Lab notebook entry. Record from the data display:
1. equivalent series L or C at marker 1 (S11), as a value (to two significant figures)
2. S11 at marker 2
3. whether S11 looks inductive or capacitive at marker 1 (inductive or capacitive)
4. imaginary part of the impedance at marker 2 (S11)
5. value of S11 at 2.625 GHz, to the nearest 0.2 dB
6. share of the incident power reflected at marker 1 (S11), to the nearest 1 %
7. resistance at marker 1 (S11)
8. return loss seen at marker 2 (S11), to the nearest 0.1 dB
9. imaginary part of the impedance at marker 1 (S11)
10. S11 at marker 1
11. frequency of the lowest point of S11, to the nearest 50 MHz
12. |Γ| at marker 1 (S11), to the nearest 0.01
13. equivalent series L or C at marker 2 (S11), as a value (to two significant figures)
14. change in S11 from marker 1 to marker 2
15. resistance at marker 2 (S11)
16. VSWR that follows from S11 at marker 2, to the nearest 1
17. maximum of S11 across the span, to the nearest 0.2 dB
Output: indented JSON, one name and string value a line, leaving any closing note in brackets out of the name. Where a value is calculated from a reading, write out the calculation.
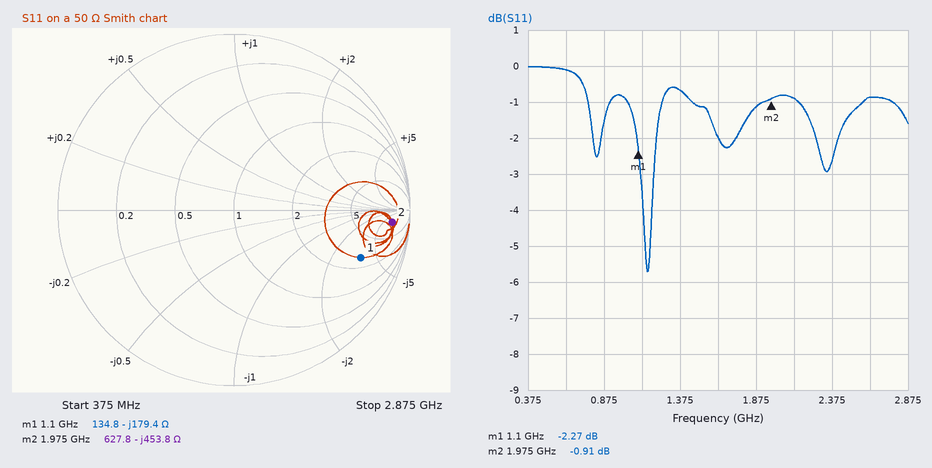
{
  "equivalent series L or C at marker 1 (S11), as a value": "C = 1/(2π × 1.1 GHz × 179.4 Ω) ≈ 807 fF, so 810 fF to two significant figures",
  "S11 at marker 2": "-0.91 dB",
  "whether S11 looks inductive or capacitive at marker 1": "capacitive",
  "imaginary part of the impedance at marker 2": "-453.8 Ω",
  "value of S11 at 2.625 GHz, to the nearest 0.2 dB": "-0.8 dB",
  "share of the incident power reflected at marker 1 (S11), to the nearest 1 %": "10^(-2.27/10) ≈ 59 %",
  "resistance at marker 1": "134.8 Ω",
  "return loss seen at marker 2 (S11), to the nearest 0.1 dB": "0.9 dB",
  "imaginary part of the impedance at marker 1": "-179.4 Ω",
  "S11 at marker 1": "-2.27 dB",
  "frequency of the lowest point of S11, to the nearest 50 MHz": "1.15 GHz",
  "|Γ| at marker 1 (S11), to the nearest 0.01": "0.77",
  "equivalent series L or C at marker 2 (S11), as a value": "C = 1/(2π × 1.975 GHz × 453.8 Ω) ≈ 178 fF, so 180 fF to two significant figures",
  "change in S11 from marker 1 to marker 2": "-0.91 − (-2.27) = 1.36 dB",
  "resistance at marker 2": "627.8 Ω",
  "VSWR that follows from S11 at marker 2, to the nearest 1": "(1 + 0.9005)/(1 − 0.9005) ≈ 19",
  "maximum of S11 across the span, to the nearest 0.2 dB": "0.0 dB"
}
